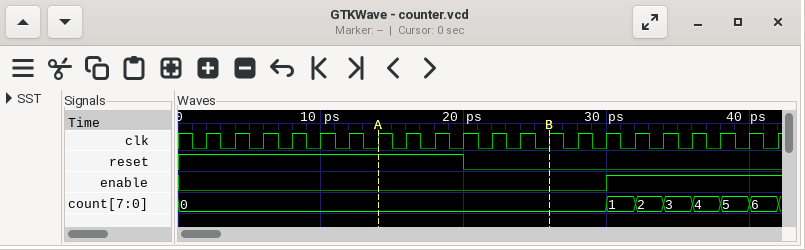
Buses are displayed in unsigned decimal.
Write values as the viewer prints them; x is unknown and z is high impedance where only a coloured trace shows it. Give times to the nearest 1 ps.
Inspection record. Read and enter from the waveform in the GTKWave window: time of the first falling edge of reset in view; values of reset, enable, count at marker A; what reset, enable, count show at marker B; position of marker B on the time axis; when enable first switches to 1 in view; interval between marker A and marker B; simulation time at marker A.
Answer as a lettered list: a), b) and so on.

a) 20 ps
b) reset=1, enable=0, count=0
c) reset=0, enable=0, count=0
d) 26 ps
e) 30 ps
f) 12 ps
g) 14 ps
